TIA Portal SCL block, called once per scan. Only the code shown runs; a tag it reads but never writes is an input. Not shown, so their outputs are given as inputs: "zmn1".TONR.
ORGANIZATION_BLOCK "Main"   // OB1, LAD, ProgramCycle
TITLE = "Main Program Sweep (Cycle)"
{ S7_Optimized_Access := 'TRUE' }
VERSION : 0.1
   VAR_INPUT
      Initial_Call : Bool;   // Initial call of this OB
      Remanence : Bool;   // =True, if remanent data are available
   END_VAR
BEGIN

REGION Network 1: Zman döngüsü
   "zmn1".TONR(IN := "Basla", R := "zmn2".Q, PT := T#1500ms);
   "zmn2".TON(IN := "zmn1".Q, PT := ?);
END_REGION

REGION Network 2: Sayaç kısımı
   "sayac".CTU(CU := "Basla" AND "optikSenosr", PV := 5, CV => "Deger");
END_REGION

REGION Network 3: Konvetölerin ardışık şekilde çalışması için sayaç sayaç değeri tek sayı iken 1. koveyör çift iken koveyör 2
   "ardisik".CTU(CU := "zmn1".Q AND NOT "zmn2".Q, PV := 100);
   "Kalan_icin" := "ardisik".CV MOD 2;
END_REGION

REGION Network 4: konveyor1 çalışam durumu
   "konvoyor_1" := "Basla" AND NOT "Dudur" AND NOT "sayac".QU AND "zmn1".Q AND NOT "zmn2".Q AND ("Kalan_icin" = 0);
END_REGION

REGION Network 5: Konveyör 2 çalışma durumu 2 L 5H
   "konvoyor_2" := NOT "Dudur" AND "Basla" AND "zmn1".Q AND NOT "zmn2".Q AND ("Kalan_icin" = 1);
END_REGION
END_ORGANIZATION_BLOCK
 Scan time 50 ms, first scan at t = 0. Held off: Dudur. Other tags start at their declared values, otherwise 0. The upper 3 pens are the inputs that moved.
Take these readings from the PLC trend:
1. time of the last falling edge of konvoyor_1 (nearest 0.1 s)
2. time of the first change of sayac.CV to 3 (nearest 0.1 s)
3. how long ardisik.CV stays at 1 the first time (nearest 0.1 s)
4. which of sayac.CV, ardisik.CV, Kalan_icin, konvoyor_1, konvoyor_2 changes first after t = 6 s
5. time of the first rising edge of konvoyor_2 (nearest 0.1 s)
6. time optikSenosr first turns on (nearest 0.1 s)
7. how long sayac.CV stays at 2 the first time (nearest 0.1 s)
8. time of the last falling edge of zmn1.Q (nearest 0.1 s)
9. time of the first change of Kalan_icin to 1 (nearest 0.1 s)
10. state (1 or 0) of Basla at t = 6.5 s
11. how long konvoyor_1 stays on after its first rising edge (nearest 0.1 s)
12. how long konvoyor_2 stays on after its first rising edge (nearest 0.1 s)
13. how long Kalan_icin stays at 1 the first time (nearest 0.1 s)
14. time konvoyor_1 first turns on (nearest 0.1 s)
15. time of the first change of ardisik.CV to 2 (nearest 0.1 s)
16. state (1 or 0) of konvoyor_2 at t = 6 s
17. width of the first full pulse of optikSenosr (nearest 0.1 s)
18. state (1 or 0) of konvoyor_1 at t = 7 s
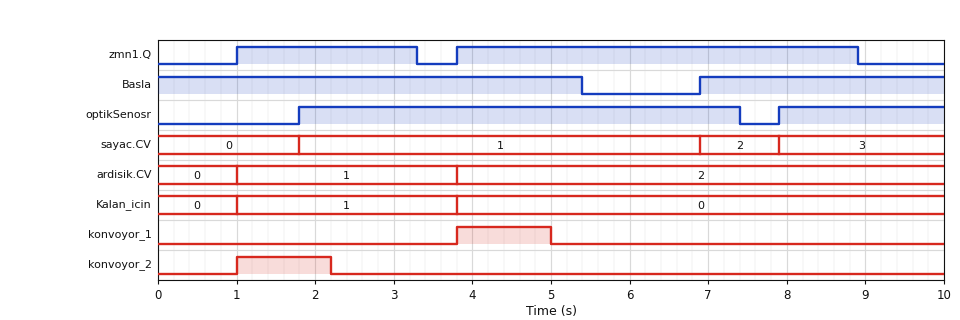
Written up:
5.0 s
7.9 s
2.8 s
sayac.CV
1.0 s
1.8 s
1.0 s
8.9 s
1.0 s
0
1.2 s
1.2 s
2.8 s
3.8 s
3.8 s
0
5.6 s
0
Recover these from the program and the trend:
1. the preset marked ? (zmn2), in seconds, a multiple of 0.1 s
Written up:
1.2 s
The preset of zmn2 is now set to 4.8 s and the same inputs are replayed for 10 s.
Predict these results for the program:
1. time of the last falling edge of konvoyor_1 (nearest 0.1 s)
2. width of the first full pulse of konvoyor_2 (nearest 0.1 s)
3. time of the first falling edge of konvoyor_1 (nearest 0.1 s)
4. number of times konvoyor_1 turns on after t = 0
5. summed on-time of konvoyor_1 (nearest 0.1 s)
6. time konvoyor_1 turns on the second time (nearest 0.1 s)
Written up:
8.6 s
2.3 s
5.4 s
2
3.3 s
6.9 s
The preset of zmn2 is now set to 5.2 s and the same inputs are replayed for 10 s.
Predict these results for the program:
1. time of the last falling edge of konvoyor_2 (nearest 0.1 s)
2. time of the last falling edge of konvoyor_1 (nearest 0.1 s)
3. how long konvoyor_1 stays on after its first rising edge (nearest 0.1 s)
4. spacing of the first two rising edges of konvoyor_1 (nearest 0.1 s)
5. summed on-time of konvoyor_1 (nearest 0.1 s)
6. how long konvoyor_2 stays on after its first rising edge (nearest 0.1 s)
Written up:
3.3 s
8.9 s
1.6 s
3.1 s
3.6 s
2.3 s
